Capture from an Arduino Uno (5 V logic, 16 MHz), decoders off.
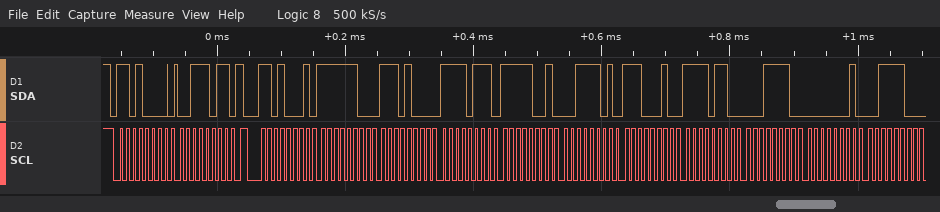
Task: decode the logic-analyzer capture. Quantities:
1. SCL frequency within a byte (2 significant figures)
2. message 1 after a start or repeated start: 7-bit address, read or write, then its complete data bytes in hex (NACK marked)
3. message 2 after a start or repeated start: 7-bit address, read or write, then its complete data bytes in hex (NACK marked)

100 kHz
0x68 write: 3B
0x68 read: FC E8 F7 F9 3D E2 F6 1E 01 3C
